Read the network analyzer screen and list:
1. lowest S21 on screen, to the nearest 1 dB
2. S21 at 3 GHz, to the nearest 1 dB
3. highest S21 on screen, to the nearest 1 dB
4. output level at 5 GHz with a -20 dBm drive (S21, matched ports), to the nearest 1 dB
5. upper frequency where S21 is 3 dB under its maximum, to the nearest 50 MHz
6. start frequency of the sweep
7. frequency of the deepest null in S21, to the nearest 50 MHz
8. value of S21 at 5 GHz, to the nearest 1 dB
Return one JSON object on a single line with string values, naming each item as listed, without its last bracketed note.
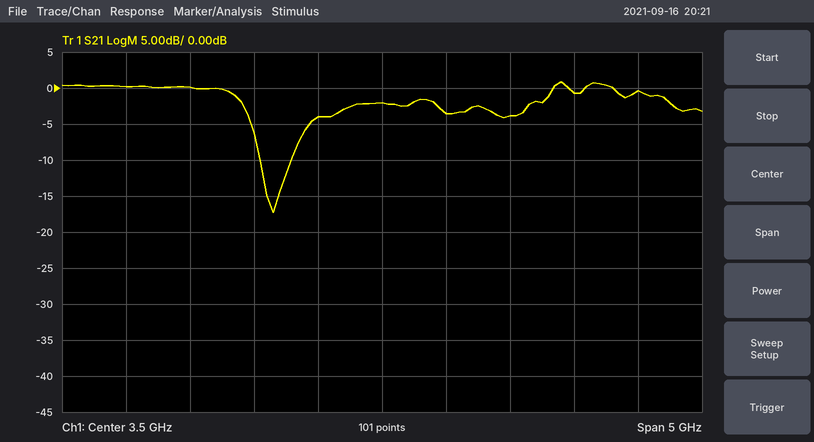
{"lowest S21 on screen, to the nearest 1 dB": "-17 dB", "S21 at 3 GHz, to the nearest 1 dB": "-4 dB", "highest S21 on screen, to the nearest 1 dB": "1 dB", "output level at 5 GHz with a -20 dBm drive (S21, matched ports), to the nearest 1 dB": "-21 dBm", "upper frequency where S21 is 3 dB under its maximum, to the nearest 50 MHz": "5.75 GHz", "start frequency of the sweep": "1 GHz", "frequency of the deepest null in S21, to the nearest 50 MHz": "2.65 GHz", "value of S21 at 5 GHz, to the nearest 1 dB": "-1 dB"}
